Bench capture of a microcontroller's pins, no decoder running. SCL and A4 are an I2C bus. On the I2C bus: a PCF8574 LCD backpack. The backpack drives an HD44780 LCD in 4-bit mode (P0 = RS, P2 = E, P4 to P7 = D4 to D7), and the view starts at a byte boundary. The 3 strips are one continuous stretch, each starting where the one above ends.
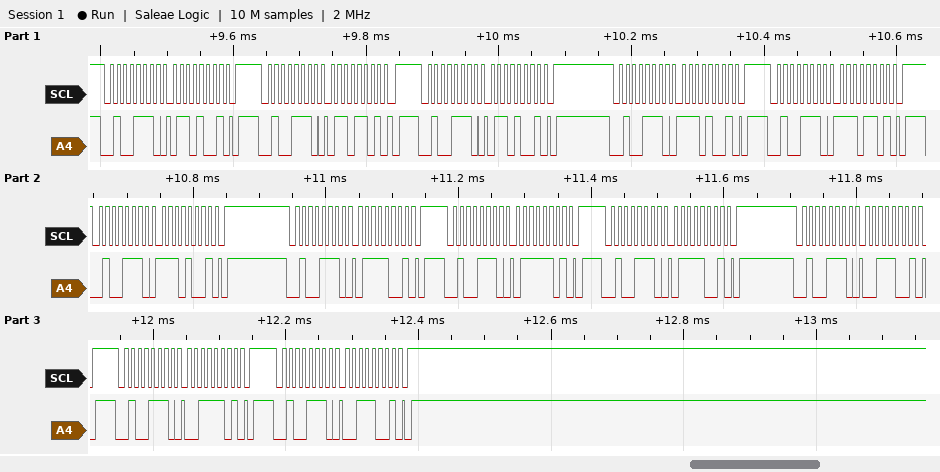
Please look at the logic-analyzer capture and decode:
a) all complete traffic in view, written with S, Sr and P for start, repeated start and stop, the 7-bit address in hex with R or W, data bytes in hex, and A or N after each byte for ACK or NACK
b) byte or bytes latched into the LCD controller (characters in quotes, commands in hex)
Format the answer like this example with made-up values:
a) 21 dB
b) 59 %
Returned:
a) S 27W A 69 A P S 27W A 6D A P S 27W A 69 A P S 27W A E9 A P S 27W A ED A P S 27W A E9 A P S 27W A 79 A P S 27W A 7D A P S 27W A 79 A P S 27W A 39 A P S 27W A 3D A P S 27W A 39 A P
b) 'n' 's'
